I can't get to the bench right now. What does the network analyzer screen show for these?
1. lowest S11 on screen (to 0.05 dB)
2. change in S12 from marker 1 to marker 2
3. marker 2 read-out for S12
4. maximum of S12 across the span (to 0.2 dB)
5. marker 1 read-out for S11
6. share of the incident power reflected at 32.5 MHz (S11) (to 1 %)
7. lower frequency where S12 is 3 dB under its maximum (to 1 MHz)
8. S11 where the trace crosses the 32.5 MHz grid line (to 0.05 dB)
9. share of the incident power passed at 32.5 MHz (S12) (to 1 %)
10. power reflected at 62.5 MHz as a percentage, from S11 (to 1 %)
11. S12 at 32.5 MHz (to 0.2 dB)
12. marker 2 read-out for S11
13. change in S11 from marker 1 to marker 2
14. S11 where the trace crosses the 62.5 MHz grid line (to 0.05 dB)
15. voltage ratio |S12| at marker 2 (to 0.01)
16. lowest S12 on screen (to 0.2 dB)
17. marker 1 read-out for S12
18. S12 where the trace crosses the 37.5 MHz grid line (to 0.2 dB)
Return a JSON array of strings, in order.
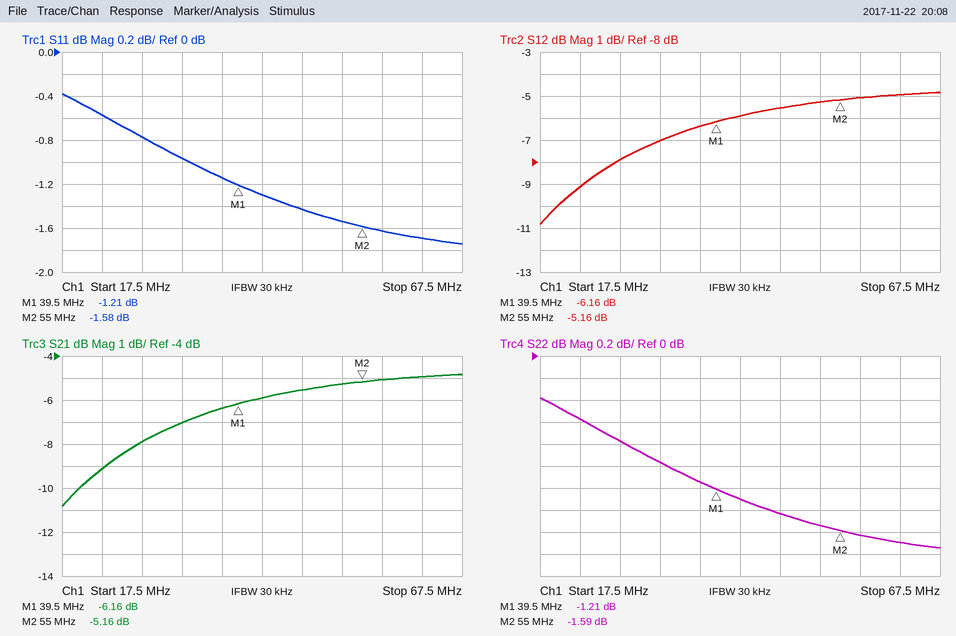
["-1.75 dB", "1.00 dB", "-5.16 dB", "-4.8 dB", "-1.21 dB", "80 %", "28 MHz", "-0.95 dB", "20 %", "68 %", "-7.0 dB", "-1.58 dB", "-0.37 dB", "-1.70 dB", "0.55", "-10.8 dB", "-6.16 dB", "-6.4 dB"]
